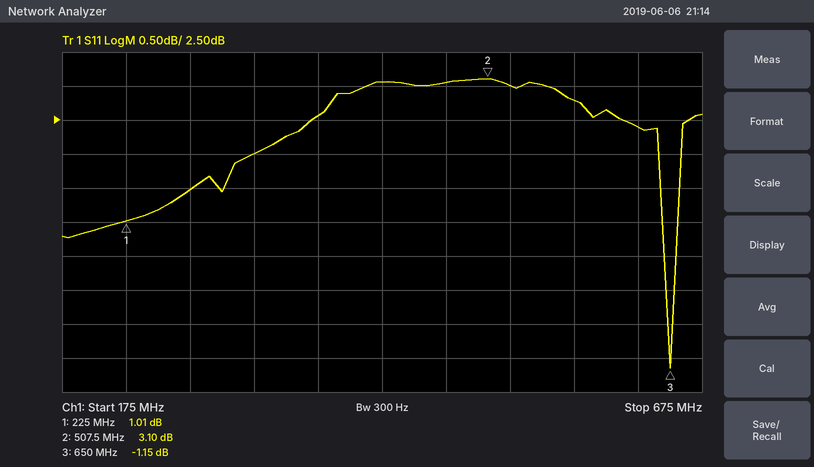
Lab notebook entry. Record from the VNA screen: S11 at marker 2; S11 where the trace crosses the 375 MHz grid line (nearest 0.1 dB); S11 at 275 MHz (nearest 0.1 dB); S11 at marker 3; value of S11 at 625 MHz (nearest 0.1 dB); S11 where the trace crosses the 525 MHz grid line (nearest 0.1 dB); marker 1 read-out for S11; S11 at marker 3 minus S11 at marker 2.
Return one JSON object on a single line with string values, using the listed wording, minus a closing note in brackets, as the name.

{"S11 at marker 2": "3.10 dB", "S11 where the trace crosses the 375 MHz grid line": "2.6 dB", "S11 at 275 MHz": "1.5 dB", "S11 at marker 3": "-1.15 dB", "value of S11 at 625 MHz": "2.4 dB", "S11 where the trace crosses the 525 MHz grid line": "3.0 dB", "marker 1 read-out for S11": "1.01 dB", "S11 at marker 3 minus S11 at marker 2": "-4.25 dB"}
